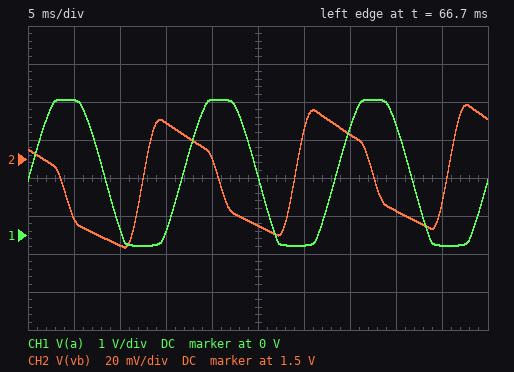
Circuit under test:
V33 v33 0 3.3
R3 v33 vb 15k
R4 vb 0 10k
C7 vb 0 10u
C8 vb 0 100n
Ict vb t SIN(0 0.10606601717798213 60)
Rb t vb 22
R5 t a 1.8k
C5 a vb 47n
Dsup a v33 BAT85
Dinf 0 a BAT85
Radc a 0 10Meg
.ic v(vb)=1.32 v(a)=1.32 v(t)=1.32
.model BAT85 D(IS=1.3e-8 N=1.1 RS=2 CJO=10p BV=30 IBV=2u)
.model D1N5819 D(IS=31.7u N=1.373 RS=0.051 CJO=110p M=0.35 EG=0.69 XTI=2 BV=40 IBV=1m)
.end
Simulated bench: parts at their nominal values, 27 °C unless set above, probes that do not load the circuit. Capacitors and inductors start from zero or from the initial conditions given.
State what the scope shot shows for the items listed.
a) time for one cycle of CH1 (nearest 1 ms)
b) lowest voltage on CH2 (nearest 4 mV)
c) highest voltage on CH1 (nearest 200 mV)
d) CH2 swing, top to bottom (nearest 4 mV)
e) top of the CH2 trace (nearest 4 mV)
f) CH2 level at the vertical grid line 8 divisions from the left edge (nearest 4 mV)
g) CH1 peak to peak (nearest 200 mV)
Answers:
17 ms
1.452 V
3.6 V
76 mV
1.528 V
1.472 V
3.8 V
